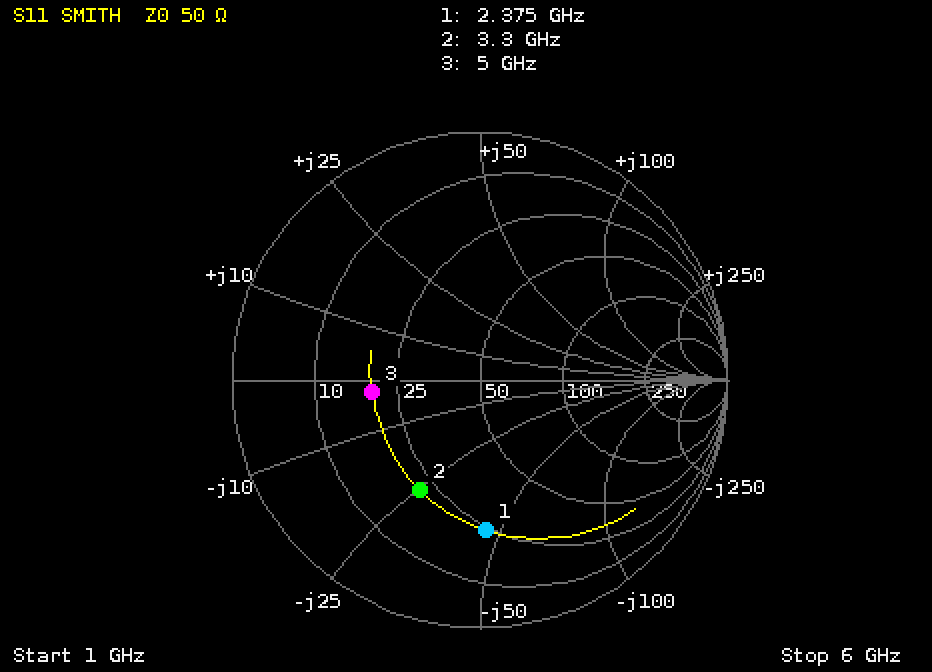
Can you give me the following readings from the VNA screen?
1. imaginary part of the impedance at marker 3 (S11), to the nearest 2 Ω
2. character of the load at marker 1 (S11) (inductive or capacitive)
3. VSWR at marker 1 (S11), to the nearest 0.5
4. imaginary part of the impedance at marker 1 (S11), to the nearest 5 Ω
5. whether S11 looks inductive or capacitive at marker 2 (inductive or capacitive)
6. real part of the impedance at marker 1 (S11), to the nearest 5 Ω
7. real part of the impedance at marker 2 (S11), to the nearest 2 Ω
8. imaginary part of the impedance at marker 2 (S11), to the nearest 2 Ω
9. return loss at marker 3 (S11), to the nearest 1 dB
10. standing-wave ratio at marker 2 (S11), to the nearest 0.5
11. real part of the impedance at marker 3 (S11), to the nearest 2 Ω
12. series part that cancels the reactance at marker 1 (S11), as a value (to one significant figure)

-2 Ω
capacitive
4.0
-45 Ω
capacitive
25 Ω
22 Ω
-26 Ω
7 dB
3.0
20 Ω
3 nH
